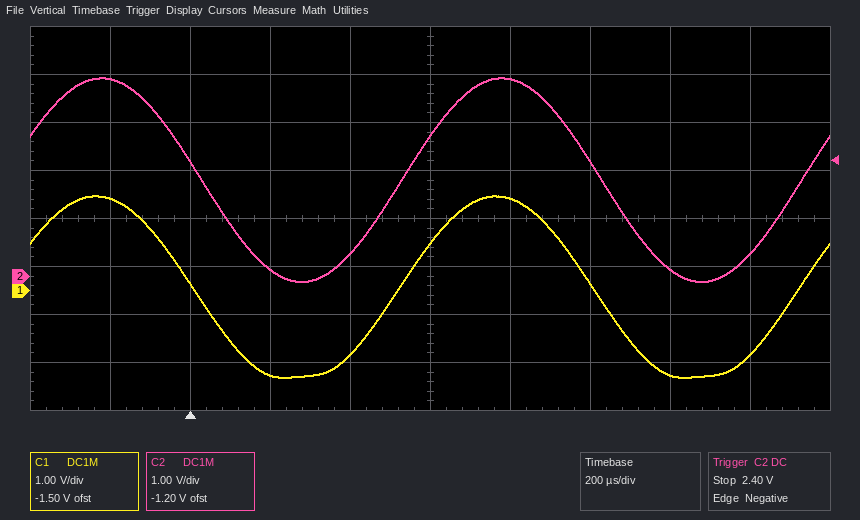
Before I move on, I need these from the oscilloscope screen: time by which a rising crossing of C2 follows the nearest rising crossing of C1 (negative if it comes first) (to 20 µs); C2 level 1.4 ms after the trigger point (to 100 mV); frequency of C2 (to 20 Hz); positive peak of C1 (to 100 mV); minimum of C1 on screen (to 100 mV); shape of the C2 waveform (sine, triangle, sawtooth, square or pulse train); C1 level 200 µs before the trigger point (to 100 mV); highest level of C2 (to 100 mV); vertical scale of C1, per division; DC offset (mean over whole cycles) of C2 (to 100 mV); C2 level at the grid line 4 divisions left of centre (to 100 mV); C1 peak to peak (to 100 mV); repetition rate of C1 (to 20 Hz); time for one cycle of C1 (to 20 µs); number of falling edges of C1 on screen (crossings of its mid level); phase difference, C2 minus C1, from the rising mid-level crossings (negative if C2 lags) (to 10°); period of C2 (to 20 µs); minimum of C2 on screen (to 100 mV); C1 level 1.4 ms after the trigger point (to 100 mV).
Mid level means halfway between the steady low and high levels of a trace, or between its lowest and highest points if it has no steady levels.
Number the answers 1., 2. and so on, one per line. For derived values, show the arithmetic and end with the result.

1. 0 µs
2. 500 mV
3. 1 / 1.00 ms ≈ 1.00 kHz
4. 2.0 V
5. -1.8 V
6. sine
7. 1.9 V
8. 4.1 V
9. 1 V
10. (4.1 V + (-100 mV)) / 2 ≈ 2.0 V
11. 4.1 V
12. 2.0 V − (-1.8 V) = 3.8 V
13. 1 / 1.00 ms ≈ 1.00 kHz
14. 1.00 ms
15. 2
16. −360° × (0 µs) / 1.00 ms ≈ 0°
17. 1.00 ms
18. -100 mV
19. -1.3 V
